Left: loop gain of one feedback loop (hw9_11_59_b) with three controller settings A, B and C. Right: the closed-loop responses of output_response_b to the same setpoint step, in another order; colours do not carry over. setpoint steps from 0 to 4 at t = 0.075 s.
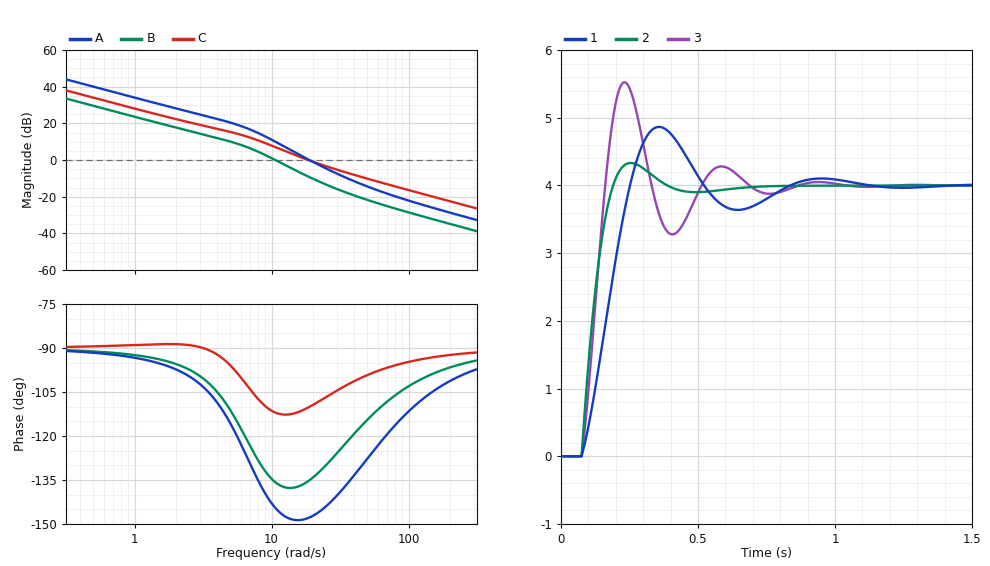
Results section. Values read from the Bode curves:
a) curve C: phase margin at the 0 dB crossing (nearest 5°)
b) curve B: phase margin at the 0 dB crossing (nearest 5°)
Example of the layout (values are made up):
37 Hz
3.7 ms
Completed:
70°
45°
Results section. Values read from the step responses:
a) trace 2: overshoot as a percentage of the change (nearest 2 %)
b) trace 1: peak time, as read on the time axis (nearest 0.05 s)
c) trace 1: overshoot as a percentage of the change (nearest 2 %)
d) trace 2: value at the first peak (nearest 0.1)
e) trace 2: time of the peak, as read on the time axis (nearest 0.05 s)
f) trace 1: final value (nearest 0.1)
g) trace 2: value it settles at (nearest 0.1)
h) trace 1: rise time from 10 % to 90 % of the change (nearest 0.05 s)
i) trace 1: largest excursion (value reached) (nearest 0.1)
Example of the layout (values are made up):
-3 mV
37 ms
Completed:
8 %
0.35 s
22 %
4.3
0.25 s
4.0
4.0
0.15 s
4.9
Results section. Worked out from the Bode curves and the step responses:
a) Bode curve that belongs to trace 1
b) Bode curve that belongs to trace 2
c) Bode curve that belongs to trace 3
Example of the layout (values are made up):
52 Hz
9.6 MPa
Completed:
B
C
A
